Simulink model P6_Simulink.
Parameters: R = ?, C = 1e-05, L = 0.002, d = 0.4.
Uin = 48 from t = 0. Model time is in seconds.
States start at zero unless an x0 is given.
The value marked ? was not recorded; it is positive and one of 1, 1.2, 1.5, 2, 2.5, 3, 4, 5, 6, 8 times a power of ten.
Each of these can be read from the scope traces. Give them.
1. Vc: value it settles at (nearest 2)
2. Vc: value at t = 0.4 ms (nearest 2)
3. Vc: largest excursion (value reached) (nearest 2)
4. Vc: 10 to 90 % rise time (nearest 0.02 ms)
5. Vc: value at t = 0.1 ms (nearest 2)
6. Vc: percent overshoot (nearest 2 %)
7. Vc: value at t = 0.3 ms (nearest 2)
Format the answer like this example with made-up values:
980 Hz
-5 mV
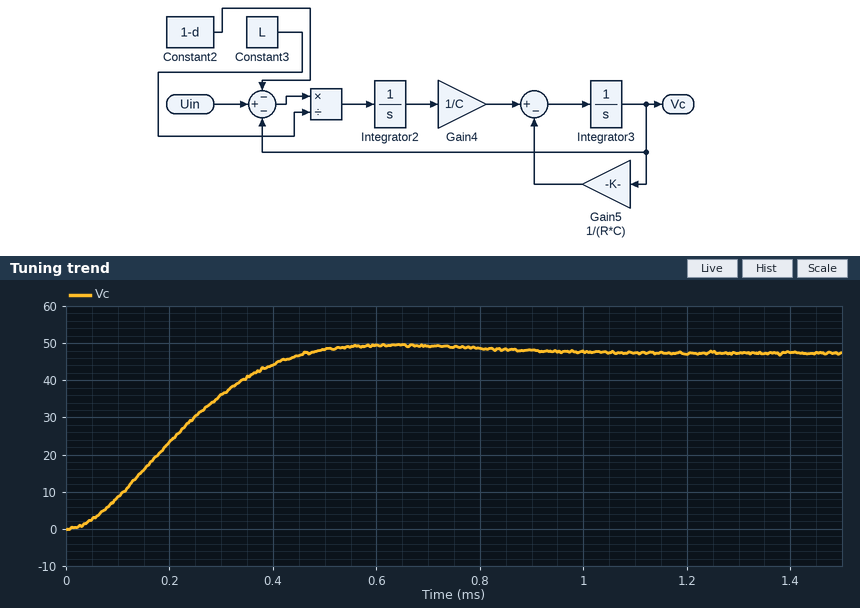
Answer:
48
44
50
0.30 ms
8
4 %
36
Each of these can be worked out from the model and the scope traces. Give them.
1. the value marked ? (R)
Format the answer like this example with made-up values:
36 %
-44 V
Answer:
10
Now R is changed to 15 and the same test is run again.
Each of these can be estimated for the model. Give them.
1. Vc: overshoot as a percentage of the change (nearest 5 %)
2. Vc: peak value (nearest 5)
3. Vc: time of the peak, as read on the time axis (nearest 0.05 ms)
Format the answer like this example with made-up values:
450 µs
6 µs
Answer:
20 %
55
0.50 ms
